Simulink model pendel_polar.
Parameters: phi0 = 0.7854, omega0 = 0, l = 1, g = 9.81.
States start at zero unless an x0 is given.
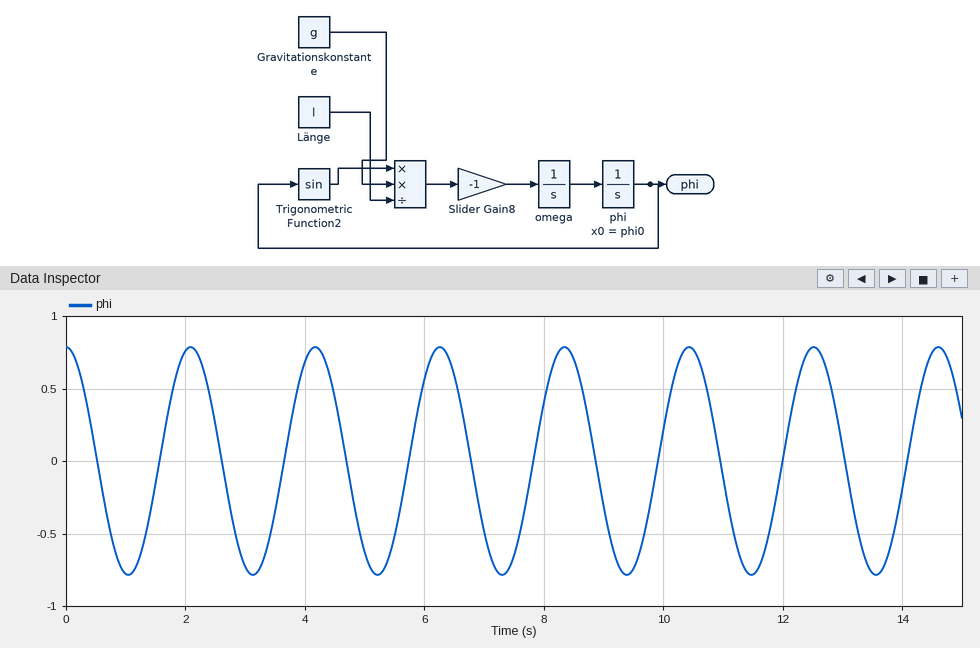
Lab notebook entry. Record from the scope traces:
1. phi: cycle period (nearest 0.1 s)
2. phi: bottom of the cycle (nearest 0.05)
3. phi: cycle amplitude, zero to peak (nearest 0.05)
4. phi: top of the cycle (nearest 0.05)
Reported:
2.1 s
-0.80
0.80
0.80
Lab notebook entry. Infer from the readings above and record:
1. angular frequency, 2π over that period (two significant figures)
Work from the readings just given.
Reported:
3.0 rad/s
